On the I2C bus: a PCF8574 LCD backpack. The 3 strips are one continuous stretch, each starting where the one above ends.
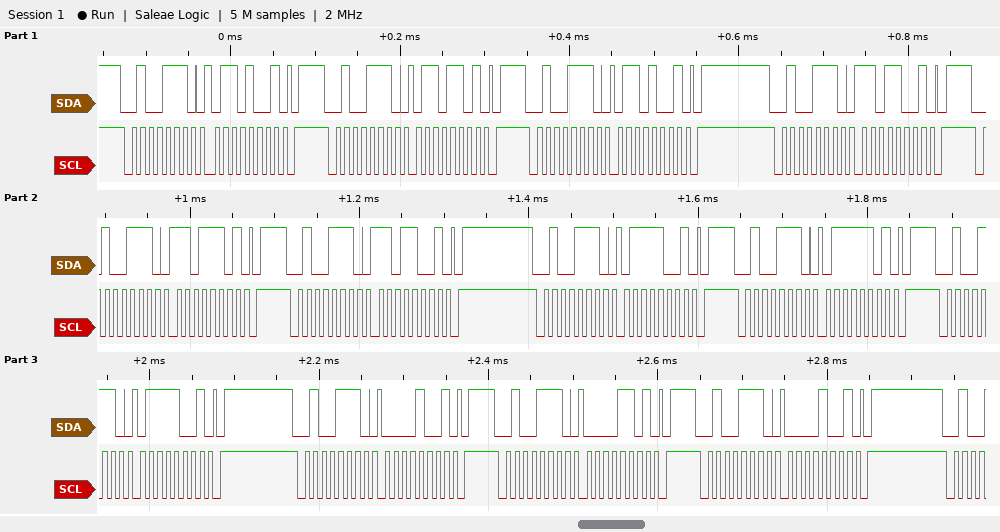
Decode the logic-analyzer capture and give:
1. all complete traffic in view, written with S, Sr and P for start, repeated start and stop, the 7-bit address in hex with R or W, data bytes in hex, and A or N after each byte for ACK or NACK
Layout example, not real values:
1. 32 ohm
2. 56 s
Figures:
1. S 27W A 69 A P S 27W A 6D A P S 27W A 69 A P S 27W A D9 A P S 27W A DD A P S 27W A D9 A P S 27W A 79 A P S 27W A 7D A P S 27W A 79 A P S 27W A 09 A P S 27W A 0D A P S 27W A 09 A P
